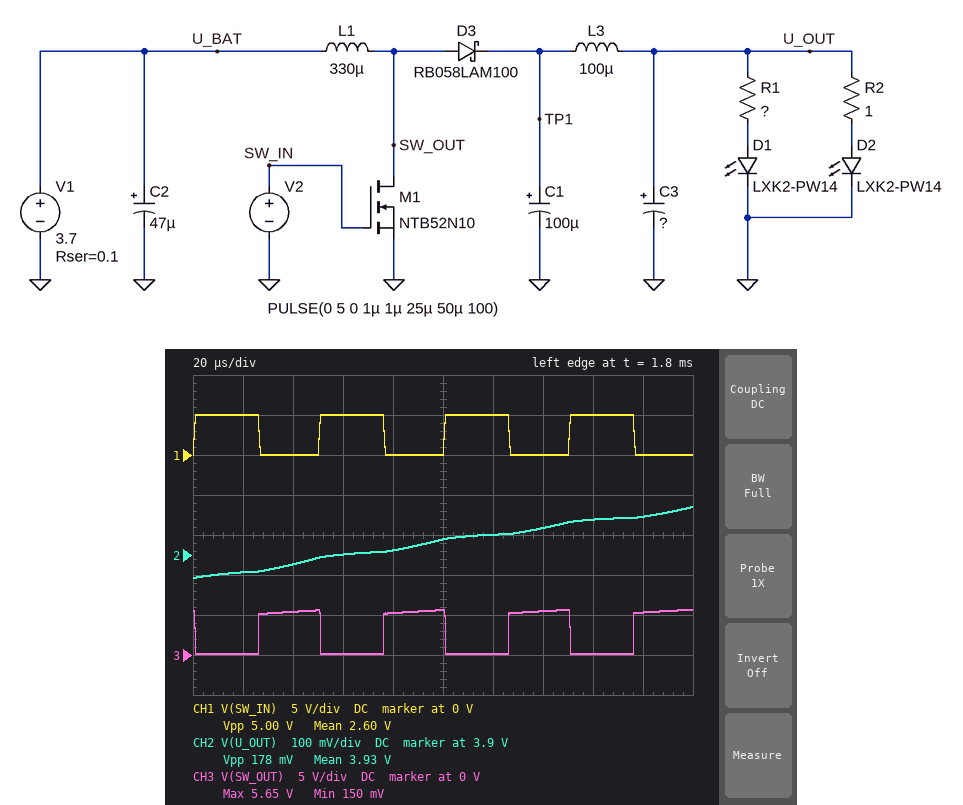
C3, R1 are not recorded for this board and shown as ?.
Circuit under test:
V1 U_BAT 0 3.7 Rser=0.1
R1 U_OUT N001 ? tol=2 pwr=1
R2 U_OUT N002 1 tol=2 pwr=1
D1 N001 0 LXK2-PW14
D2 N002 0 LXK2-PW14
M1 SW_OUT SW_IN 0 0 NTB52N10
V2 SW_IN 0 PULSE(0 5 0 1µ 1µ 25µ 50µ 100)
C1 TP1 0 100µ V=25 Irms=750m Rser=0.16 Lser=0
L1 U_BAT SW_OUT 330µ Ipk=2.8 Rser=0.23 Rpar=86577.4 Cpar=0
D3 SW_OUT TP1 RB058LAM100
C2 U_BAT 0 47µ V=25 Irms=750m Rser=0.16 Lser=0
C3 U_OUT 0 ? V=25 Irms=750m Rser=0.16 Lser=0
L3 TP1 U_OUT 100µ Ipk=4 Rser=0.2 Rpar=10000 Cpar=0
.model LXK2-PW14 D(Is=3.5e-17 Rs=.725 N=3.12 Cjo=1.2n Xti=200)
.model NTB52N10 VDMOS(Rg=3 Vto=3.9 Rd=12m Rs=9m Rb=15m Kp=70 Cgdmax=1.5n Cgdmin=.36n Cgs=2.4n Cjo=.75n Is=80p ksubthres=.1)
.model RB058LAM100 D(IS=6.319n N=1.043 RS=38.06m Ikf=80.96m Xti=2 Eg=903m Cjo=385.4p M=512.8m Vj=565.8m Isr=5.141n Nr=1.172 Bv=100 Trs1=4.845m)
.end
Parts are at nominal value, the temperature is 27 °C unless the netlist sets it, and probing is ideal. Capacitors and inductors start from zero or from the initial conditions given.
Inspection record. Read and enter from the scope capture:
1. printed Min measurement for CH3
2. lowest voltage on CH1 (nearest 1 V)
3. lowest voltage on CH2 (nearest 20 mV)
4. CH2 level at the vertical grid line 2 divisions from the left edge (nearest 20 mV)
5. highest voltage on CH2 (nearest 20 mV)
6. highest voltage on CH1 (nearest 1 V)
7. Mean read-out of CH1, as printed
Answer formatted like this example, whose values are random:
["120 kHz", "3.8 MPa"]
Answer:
["150 mV", "0 V", "3.84 V", "3.88 V", "4.02 V", "5 V", "2.60 V"]
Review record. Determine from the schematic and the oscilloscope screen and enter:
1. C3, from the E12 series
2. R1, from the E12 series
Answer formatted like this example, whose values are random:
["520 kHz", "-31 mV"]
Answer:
["680 µF", "0.82 Ω"]
